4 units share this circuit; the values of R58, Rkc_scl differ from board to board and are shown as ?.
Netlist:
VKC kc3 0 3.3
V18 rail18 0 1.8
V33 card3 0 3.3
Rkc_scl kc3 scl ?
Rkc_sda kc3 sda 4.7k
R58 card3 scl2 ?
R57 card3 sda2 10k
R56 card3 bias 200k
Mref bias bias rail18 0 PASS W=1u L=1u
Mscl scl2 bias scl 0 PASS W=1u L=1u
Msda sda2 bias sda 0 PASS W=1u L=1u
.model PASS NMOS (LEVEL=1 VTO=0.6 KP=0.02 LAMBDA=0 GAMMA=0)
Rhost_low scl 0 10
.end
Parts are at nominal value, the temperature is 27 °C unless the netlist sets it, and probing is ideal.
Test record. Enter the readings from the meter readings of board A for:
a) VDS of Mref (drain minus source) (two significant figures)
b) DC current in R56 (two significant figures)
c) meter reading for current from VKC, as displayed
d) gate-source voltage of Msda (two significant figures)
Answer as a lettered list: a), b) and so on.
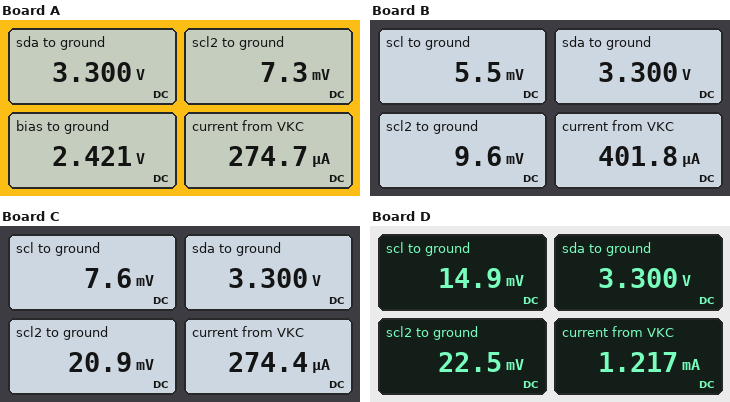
a) 620 mV
b) 4.4 µA
c) 274.7 µA
d) -880 mV
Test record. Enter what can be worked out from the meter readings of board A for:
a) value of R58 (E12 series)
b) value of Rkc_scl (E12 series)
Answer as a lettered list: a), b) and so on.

a) 27 kΩ
b) 12 kΩ
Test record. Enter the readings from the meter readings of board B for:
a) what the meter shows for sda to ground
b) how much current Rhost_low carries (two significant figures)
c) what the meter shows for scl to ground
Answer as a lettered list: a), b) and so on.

a) 3.300 V
b) 550 µA
c) 5.5 mV
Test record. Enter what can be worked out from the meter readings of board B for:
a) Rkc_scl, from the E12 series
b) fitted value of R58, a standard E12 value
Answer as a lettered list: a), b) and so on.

a) 8.2 kΩ
b) 22 kΩ
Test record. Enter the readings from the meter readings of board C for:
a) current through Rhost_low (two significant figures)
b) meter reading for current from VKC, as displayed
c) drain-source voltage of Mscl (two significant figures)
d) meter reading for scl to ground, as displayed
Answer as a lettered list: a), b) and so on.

a) 760 µA
b) 274.4 µA
c) 13 mV
d) 7.6 mV
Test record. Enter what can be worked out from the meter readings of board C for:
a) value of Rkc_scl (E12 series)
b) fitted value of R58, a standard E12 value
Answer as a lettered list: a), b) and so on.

a) 12 kΩ
b) 6.8 kΩ
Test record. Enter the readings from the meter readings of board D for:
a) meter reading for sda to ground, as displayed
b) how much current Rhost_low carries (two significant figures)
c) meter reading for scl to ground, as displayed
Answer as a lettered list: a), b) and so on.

a) 3.300 V
b) 1.5 mA
c) 14.9 mV
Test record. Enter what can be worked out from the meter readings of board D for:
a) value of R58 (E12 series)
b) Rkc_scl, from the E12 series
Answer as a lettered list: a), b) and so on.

a) 12 kΩ
b) 2.7 kΩ
